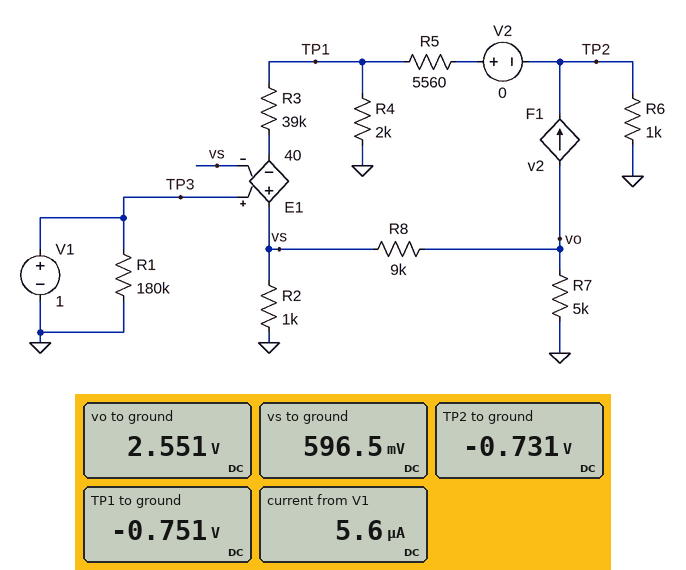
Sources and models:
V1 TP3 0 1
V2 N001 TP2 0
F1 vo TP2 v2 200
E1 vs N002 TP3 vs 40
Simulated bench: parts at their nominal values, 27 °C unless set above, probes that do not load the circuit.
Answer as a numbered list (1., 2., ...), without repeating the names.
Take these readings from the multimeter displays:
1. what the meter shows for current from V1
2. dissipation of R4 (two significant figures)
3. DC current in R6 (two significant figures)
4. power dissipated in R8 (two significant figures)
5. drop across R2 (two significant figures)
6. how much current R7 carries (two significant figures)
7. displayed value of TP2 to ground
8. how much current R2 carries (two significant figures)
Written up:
1. 5.6 µA
2. 280 µW
3. 730 µA
4. 420 µW
5. 600 mV
6. 510 µA
7. -0.731 V
8. 600 µA
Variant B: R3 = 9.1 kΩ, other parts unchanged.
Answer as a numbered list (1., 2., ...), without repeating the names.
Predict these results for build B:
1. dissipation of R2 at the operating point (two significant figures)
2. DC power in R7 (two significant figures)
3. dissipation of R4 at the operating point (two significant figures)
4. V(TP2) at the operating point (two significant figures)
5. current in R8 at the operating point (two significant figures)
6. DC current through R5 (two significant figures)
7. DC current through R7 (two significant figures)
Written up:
1. 690 µW
2. 2.5 mW
3. 550 µW
4. -1.0 V
5. 300 µA
6. 5.1 µA
7. 710 µA
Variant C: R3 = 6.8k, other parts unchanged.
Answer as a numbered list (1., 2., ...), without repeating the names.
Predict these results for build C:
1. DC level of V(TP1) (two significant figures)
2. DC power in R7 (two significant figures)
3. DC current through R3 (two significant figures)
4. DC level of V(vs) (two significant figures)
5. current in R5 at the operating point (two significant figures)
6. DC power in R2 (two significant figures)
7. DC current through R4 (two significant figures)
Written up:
1. -1.1 V
2. 2.7 mW
3. 550 µA
4. 860 mV
5. 5.2 µA
6. 740 µW
7. 540 µA
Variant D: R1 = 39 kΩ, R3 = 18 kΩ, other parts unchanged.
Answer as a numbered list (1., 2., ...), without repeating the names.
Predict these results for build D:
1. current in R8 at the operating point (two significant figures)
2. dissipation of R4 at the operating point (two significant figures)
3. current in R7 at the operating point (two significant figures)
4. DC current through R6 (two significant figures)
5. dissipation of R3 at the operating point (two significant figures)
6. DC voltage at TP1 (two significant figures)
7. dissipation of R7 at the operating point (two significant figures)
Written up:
1. 270 µA
2. 440 µW
3. 640 µA
4. 910 µA
5. 4.0 mW
6. -940 mV
7. 2.0 mW
